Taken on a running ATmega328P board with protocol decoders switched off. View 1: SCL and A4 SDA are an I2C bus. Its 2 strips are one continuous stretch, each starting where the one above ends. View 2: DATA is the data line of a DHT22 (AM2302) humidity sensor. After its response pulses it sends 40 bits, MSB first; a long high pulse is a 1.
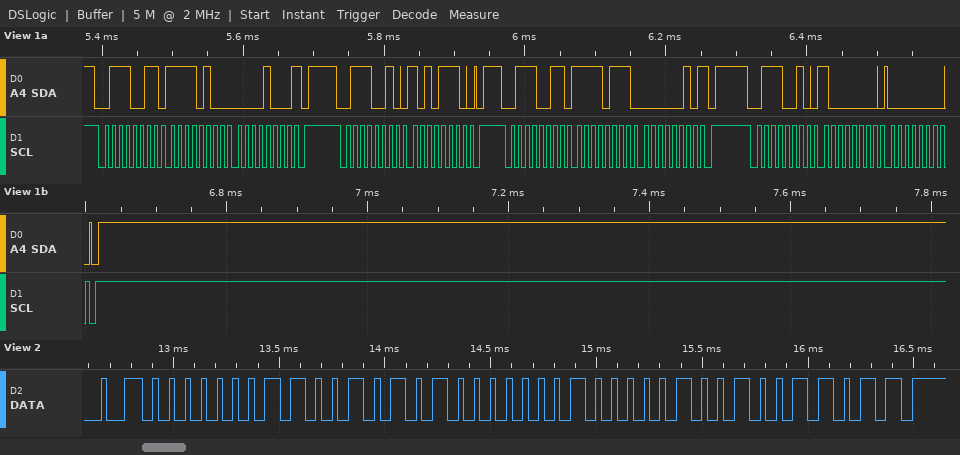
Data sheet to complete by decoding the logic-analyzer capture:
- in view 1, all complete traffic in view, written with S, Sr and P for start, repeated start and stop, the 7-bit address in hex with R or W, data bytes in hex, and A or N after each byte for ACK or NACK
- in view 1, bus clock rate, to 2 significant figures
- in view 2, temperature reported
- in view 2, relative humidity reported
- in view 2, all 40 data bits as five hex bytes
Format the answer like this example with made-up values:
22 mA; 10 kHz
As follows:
S 39R A F4 A 08 N P S 39W A AE A P S 39R A F7 A 02 N P S 39W A 80 A 00 A P; 100 kHz; 26.0 °C; 40.5 %; 01 95 01 04 9B
